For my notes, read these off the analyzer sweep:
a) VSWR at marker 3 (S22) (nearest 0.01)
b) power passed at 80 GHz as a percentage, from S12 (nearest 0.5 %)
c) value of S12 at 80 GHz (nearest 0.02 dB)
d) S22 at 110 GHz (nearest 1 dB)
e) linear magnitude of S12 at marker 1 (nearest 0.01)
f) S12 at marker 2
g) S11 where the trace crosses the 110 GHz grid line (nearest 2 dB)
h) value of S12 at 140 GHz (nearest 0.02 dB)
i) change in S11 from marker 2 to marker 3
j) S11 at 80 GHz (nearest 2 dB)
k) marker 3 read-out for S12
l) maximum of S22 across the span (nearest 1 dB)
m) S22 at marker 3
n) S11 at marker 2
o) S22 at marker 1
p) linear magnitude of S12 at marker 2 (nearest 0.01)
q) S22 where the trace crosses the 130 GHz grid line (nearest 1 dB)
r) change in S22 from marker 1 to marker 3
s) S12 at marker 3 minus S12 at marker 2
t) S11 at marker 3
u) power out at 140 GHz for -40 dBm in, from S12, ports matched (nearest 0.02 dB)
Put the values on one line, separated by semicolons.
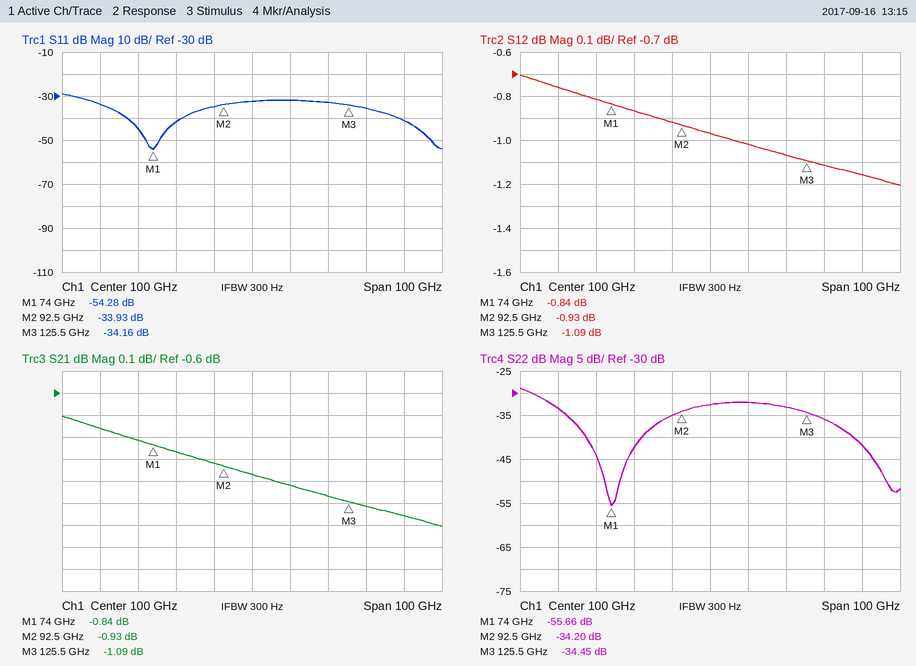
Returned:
1.04; 82.0 %; -0.86 dB; -32 dB; 0.91; -0.93 dB; -32 dB; -1.16 dB; -0.23 dB; -42 dB; -1.09 dB; -29 dB; -34.45 dB; -33.93 dB; -55.66 dB; 0.90; -36 dB; 21.21 dB; -0.16 dB; -34.16 dB; -41.16 dBm
